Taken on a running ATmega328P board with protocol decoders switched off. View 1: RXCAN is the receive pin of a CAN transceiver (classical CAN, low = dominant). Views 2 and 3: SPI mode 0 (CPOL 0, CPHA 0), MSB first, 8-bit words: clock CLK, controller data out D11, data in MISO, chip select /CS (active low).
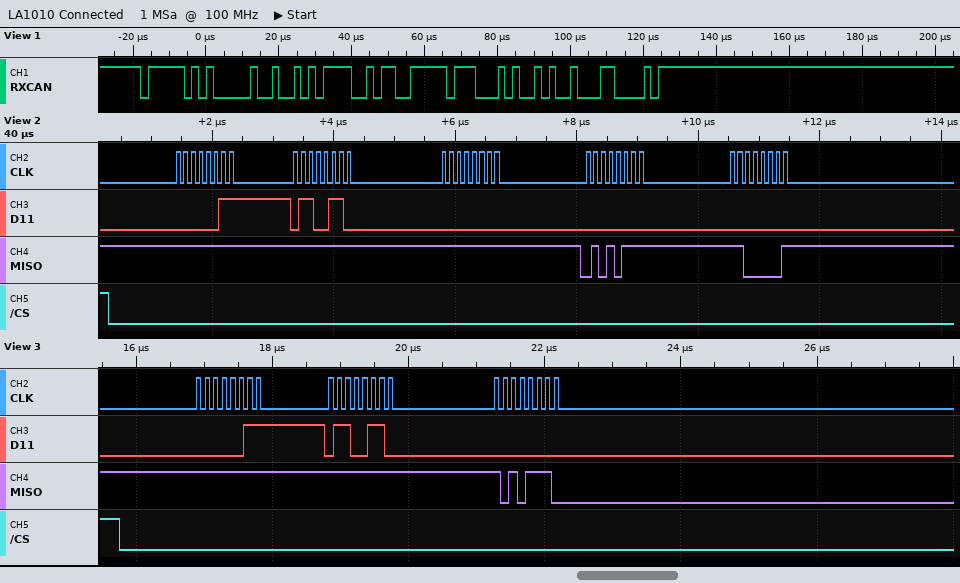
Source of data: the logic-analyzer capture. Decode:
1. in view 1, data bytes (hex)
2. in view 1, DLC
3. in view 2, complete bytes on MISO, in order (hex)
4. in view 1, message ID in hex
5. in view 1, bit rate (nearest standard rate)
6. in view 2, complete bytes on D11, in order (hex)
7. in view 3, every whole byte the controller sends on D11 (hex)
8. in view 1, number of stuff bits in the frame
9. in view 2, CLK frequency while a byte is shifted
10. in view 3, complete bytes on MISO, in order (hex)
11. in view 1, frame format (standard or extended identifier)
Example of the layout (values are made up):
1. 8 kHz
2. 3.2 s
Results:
1. AF 2C FF 14
2. 4
3. 0xFF 0xFF 0xFF 0x57 0xC1
4. 0x7E8
5. 500 kbit/s
6. 0x03 0x66 0x00 0x00 0x00
7. 03 66 00
8. 3
9. 8 MHz
10. FF FF AE
11. standard
